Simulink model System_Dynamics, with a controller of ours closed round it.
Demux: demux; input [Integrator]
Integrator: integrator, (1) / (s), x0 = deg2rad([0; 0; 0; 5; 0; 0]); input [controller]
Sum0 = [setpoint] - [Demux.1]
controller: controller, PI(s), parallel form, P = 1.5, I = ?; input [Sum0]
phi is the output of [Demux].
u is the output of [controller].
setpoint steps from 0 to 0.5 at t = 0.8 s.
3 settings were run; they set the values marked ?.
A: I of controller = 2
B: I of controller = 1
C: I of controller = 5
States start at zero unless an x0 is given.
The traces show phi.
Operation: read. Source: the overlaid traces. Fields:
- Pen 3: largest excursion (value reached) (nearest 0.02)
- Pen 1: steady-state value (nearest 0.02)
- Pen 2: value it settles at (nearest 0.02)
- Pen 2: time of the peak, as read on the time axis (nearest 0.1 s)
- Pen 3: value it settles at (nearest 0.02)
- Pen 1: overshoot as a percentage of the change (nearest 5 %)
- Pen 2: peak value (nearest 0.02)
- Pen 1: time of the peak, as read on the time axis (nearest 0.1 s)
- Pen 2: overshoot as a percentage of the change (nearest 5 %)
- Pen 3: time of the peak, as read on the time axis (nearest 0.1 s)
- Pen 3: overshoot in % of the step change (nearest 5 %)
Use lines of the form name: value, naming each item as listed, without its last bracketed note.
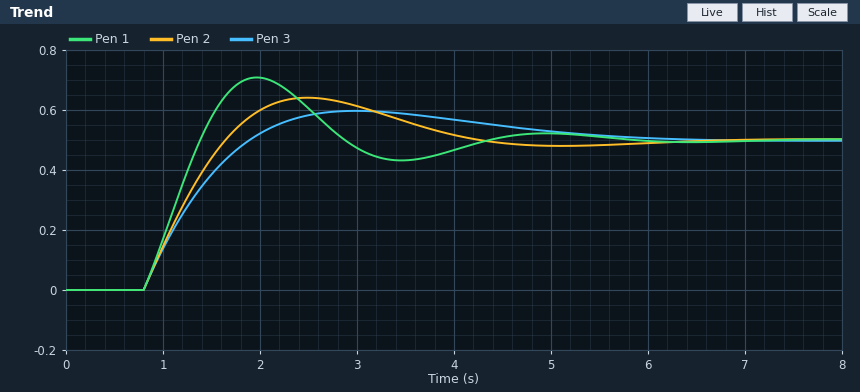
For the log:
Pen 3: largest excursion (value reached): 0.60
Pen 1: steady-state value: 0.50
Pen 2: value it settles at: 0.50
Pen 2: time of the peak, as read on the time axis: 2.5 s
Pen 3: value it settles at: 0.50
Pen 1: overshoot as a percentage of the change: 40 %
Pen 2: peak value: 0.64
Pen 1: time of the peak, as read on the time axis: 2.0 s
Pen 2: overshoot as a percentage of the change: 30 %
Pen 3: time of the peak, as read on the time axis: 3.0 s
Pen 3: overshoot in % of the step change: 20 %
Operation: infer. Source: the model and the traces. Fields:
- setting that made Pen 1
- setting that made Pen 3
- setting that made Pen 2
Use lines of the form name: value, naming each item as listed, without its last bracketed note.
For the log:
setting that made Pen 1: C
setting that made Pen 3: B
setting that made Pen 2: A
